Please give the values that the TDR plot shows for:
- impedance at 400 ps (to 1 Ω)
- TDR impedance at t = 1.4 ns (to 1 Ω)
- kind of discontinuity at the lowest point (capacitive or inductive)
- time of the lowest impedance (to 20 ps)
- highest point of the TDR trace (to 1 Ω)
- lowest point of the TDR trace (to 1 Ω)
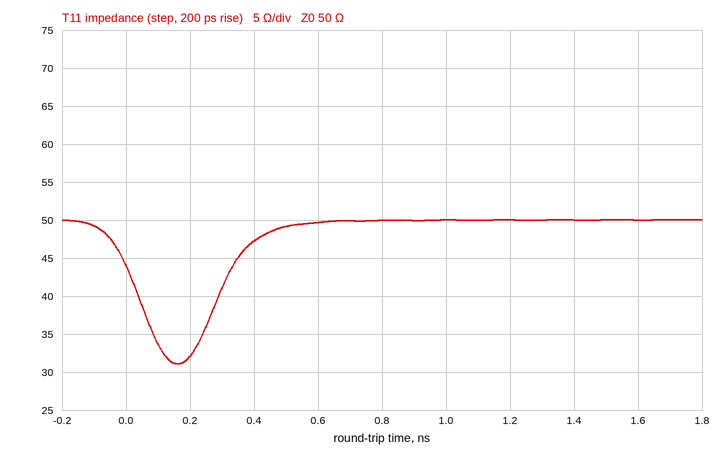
47 Ω
50 Ω
capacitive
160 ps
50 Ω
31 Ω
